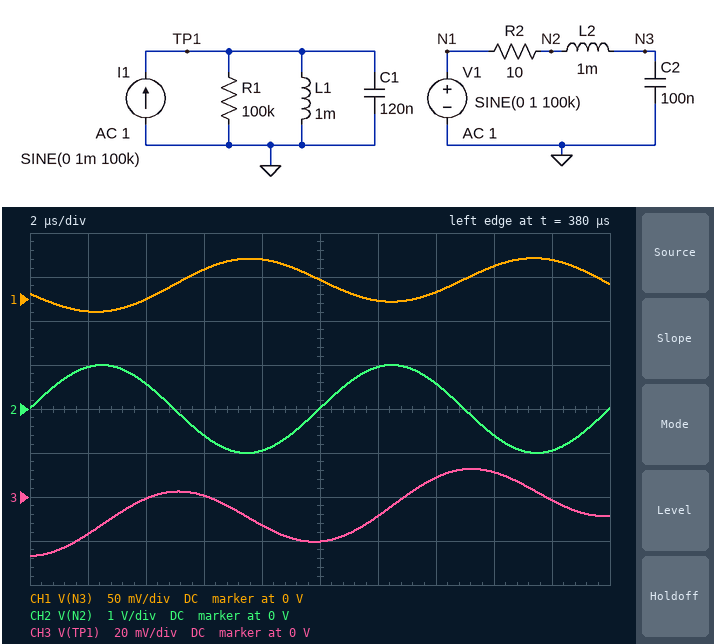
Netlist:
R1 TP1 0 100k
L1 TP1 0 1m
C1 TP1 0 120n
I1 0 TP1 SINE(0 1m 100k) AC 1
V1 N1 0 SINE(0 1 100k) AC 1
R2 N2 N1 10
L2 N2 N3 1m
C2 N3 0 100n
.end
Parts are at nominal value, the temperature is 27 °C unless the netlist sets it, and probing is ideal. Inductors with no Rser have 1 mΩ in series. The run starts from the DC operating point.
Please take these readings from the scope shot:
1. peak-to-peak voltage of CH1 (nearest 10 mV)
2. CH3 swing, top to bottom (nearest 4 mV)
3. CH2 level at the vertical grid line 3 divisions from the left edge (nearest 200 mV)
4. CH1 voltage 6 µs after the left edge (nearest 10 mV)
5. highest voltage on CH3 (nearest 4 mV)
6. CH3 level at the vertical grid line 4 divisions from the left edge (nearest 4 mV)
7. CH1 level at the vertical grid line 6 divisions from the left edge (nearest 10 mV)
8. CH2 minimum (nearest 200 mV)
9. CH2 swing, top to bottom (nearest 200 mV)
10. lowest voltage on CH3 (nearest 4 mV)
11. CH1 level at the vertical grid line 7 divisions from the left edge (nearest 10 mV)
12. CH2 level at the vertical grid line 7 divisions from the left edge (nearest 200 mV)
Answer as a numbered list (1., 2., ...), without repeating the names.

1. 60 mV
2. 40 mV
3. -600 mV
4. 30 mV
5. 12 mV
6. -12 mV
7. 0 V
8. -1.0 V
9. 2.0 V
10. -28 mV
11. 10 mV
12. 600 mV
